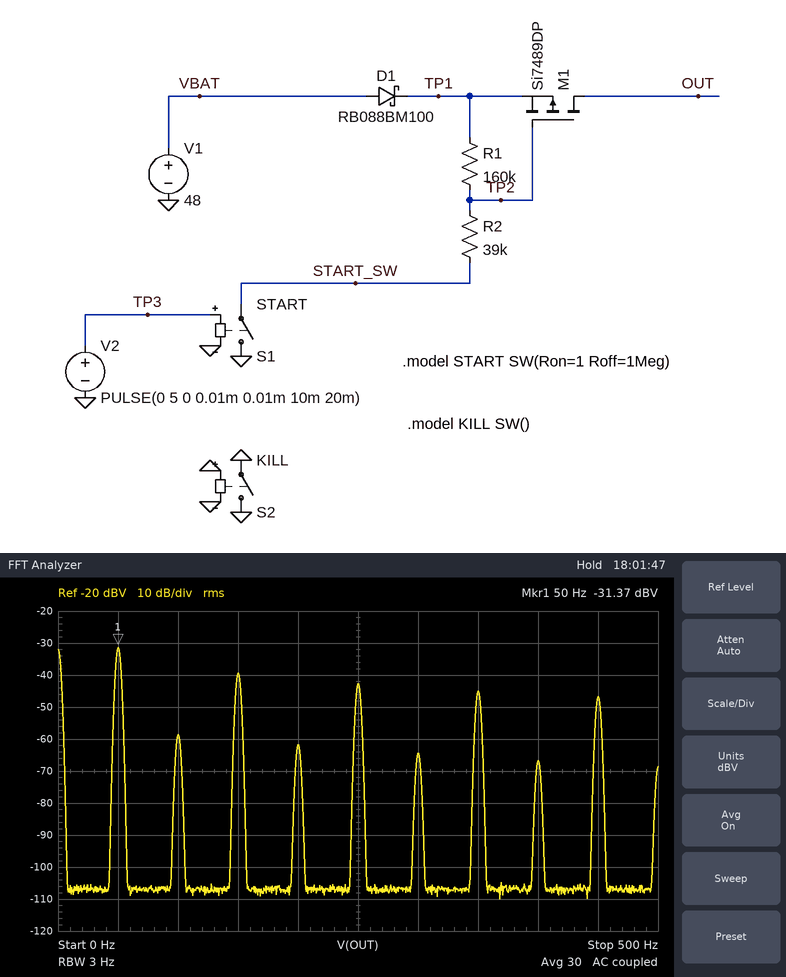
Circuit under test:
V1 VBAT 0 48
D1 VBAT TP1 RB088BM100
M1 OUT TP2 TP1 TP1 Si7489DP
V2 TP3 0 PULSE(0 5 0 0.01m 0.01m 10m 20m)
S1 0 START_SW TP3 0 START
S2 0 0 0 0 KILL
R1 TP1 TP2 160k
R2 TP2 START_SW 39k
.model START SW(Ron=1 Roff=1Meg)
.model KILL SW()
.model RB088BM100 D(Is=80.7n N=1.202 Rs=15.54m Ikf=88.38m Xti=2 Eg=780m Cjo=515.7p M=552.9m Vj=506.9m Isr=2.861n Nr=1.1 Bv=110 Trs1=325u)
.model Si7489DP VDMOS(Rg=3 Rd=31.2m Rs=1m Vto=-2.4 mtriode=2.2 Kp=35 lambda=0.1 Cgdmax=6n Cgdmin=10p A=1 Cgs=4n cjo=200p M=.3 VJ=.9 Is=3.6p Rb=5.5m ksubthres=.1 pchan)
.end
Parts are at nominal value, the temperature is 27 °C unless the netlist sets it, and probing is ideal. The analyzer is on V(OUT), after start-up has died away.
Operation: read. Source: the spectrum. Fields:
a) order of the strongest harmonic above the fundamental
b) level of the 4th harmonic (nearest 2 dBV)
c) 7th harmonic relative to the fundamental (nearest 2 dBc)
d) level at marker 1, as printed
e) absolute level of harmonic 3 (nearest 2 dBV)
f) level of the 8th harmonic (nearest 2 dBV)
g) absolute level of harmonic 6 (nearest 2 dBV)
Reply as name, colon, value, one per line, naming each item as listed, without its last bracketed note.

order of the strongest harmonic above the fundamental: 3
level of the 4th harmonic: -62 dBV
7th harmonic relative to the fundamental: -14 dBc
level at marker 1, as printed: -31.37 dBV
absolute level of harmonic 3: -40 dBV
level of the 8th harmonic: -66 dBV
absolute level of harmonic 6: -64 dBV
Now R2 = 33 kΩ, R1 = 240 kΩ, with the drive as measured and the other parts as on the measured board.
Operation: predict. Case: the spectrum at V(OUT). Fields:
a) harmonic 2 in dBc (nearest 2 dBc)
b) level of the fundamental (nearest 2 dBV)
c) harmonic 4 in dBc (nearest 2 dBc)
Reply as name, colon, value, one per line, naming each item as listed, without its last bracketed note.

harmonic 2 in dBc: -22 dBc
level of the fundamental: -32 dBV
harmonic 4 in dBc: -26 dBc
